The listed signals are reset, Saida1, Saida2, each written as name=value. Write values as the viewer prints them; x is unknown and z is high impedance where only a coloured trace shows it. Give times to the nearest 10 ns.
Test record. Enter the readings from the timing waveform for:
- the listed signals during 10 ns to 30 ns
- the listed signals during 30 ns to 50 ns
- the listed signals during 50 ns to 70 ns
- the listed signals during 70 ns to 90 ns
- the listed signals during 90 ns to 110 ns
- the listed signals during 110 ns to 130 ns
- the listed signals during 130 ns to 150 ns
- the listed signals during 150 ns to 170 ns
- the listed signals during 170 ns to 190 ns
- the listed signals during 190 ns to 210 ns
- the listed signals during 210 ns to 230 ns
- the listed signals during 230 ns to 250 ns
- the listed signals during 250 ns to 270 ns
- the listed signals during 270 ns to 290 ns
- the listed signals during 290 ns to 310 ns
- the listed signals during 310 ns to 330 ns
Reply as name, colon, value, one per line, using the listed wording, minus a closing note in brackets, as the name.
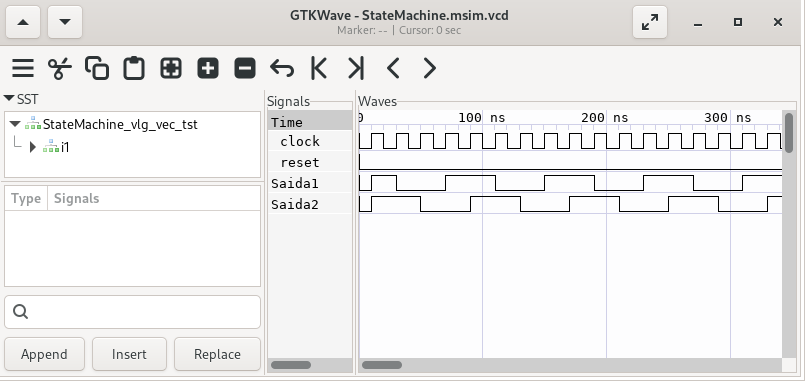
the listed signals during 10 ns to 30 ns: reset=0, Saida1=1, Saida2=1
the listed signals during 30 ns to 50 ns: reset=0, Saida1=0, Saida2=1
the listed signals during 50 ns to 70 ns: reset=0, Saida1=0, Saida2=0
the listed signals during 70 ns to 90 ns: reset=0, Saida1=1, Saida2=0
the listed signals during 90 ns to 110 ns: reset=0, Saida1=1, Saida2=1
the listed signals during 110 ns to 130 ns: reset=0, Saida1=0, Saida2=1
the listed signals during 130 ns to 150 ns: reset=0, Saida1=0, Saida2=0
the listed signals during 150 ns to 170 ns: reset=0, Saida1=1, Saida2=0
the listed signals during 170 ns to 190 ns: reset=0, Saida1=1, Saida2=1
the listed signals during 190 ns to 210 ns: reset=0, Saida1=0, Saida2=1
the listed signals during 210 ns to 230 ns: reset=0, Saida1=0, Saida2=0
the listed signals during 230 ns to 250 ns: reset=0, Saida1=1, Saida2=0
the listed signals during 250 ns to 270 ns: reset=0, Saida1=1, Saida2=1
the listed signals during 270 ns to 290 ns: reset=0, Saida1=0, Saida2=1
the listed signals during 290 ns to 310 ns: reset=0, Saida1=0, Saida2=0
the listed signals during 310 ns to 330 ns: reset=0, Saida1=1, Saida2=0
